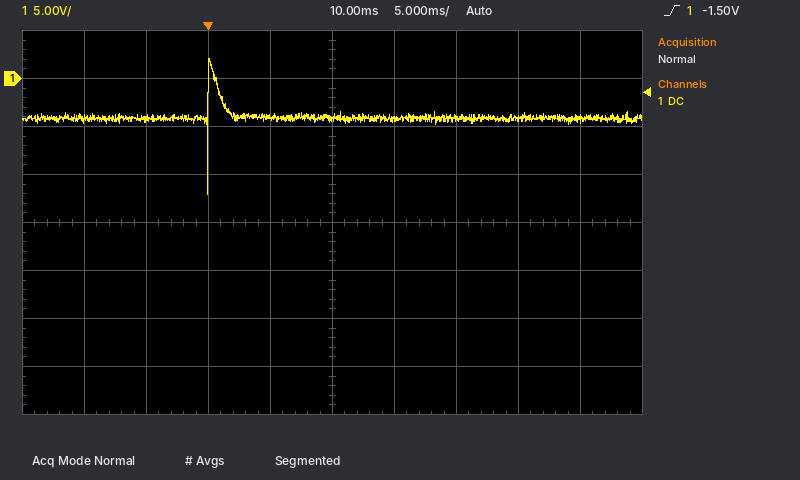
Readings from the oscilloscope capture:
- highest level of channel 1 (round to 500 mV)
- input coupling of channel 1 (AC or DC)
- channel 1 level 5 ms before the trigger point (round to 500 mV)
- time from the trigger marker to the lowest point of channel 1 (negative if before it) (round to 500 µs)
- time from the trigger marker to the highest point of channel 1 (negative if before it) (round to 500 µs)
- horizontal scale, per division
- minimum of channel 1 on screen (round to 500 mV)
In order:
2.0 V
DC
-4.0 V
0.0 ms
0.0 ms
5 ms
-12.0 V
